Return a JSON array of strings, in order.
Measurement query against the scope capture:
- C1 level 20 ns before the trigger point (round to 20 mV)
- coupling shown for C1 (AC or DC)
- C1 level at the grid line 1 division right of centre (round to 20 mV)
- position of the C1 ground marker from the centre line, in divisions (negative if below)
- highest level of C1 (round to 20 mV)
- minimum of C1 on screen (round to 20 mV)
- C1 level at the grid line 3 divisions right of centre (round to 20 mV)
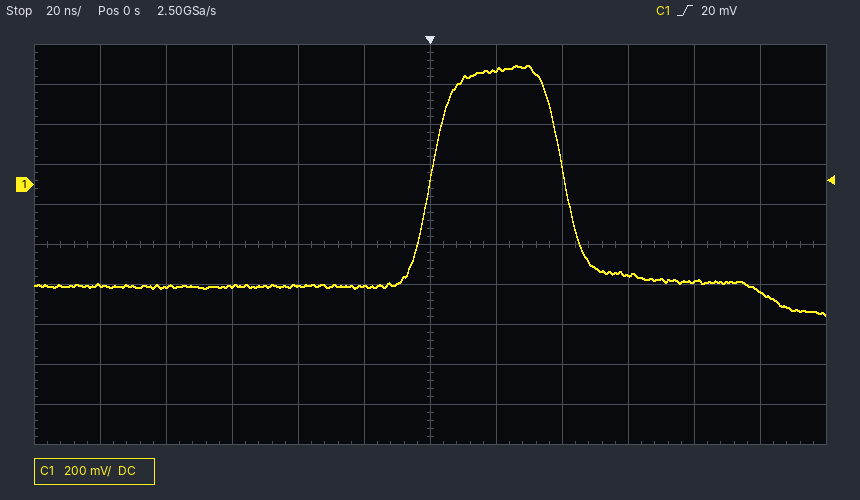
["-500 mV", "DC", "580 mV", "+1.5 div", "600 mV", "-660 mV", "-460 mV"]
